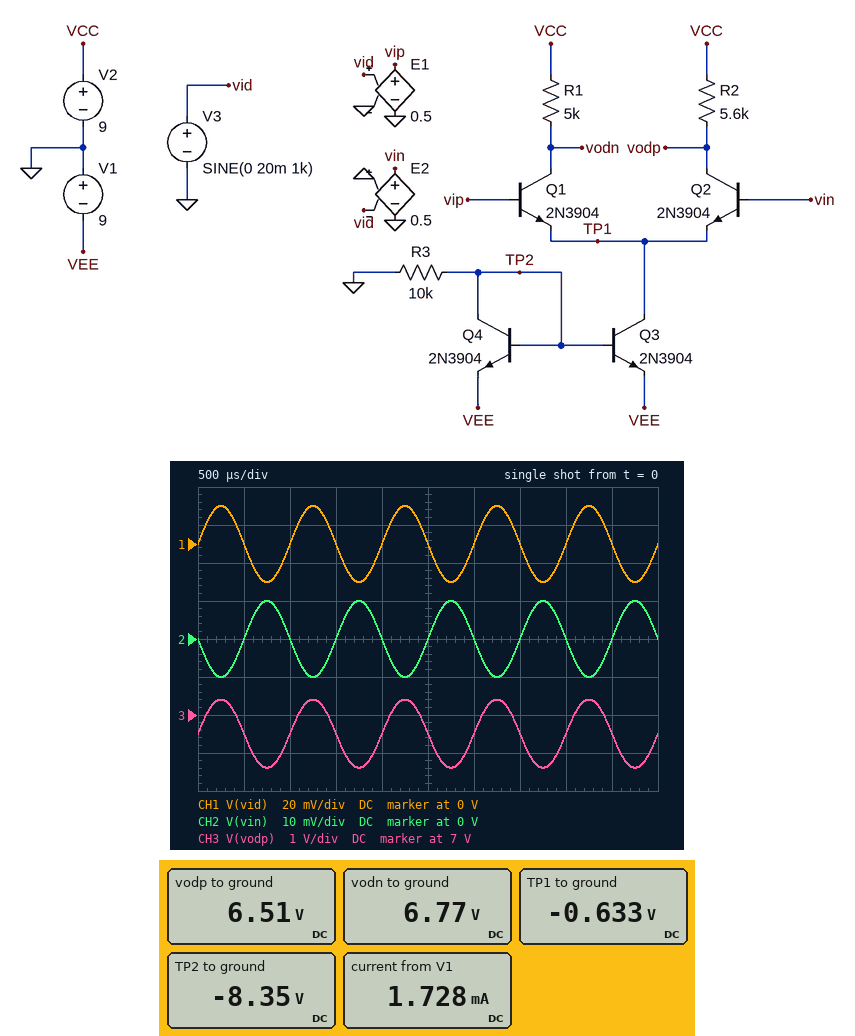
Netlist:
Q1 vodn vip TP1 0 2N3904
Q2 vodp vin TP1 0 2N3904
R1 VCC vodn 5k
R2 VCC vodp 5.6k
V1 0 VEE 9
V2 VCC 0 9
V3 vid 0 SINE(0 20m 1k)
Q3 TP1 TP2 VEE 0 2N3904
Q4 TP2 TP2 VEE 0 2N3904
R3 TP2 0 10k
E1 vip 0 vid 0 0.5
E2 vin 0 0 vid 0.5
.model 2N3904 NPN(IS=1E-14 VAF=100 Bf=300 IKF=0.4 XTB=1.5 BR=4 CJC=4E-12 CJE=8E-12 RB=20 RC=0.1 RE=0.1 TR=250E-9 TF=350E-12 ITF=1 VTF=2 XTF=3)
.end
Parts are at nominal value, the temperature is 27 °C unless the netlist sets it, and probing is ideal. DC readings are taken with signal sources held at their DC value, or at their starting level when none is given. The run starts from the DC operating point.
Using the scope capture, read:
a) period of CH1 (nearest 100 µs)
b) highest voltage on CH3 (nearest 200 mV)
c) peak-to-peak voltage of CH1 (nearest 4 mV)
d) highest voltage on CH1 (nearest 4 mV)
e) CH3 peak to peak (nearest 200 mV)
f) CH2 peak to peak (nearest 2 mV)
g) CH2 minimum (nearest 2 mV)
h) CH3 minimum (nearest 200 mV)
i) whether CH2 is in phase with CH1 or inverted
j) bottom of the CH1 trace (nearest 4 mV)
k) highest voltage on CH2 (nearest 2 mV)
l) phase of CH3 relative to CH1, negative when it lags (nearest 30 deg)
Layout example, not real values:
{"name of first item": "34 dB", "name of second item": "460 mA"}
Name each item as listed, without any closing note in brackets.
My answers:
{"period of CH1": "1.0 ms", "highest voltage on CH3": "7.4 V", "peak-to-peak voltage of CH1": "40 mV", "highest voltage on CH1": "20 mV", "CH3 peak to peak": "1.8 V", "CH2 peak to peak": "20 mV", "CH2 minimum": "-10 mV", "CH3 minimum": "5.6 V", "whether CH2 is in phase with CH1 or inverted": "inverted", "bottom of the CH1 trace": "-20 mV", "highest voltage on CH2": "10 mV", "phase of CH3 relative to CH1, negative when it lags": "0 deg"}
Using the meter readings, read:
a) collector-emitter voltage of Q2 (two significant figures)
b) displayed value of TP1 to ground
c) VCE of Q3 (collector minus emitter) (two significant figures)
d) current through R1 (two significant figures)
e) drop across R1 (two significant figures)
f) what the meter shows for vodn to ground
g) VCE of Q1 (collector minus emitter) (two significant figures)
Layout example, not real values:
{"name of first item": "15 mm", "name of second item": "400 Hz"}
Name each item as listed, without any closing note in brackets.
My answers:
{"collector-emitter voltage of Q2": "7.1 V", "displayed value of TP1 to ground": "-0.633 V", "VCE of Q3 (collector minus emitter)": "8.4 V", "current through R1": "450 µA", "drop across R1": "2.2 V", "what the meter shows for vodn to ground": "6.77 V", "VCE of Q1 (collector minus emitter)": "7.4 V"}
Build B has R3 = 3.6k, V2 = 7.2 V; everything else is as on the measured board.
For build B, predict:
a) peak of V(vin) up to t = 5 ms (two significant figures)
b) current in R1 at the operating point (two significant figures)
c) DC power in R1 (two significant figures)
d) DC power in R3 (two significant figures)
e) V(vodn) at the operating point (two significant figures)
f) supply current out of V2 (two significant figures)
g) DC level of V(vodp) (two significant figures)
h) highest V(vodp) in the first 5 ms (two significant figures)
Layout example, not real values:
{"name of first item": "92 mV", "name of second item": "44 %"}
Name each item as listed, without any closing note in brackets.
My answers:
{"peak of V(vin) up to t = 5 ms": "10 mV", "current in R1 at the operating point": "1.2 mA", "DC power in R1": "7.6 mW", "DC power in R3": "19 mW", "V(vodn) at the operating point": "1.0 V", "supply current out of V2": "2.5 mA", "DC level of V(vodp)": "330 mV", "highest V(vodp) in the first 5 ms": "2.4 V"}
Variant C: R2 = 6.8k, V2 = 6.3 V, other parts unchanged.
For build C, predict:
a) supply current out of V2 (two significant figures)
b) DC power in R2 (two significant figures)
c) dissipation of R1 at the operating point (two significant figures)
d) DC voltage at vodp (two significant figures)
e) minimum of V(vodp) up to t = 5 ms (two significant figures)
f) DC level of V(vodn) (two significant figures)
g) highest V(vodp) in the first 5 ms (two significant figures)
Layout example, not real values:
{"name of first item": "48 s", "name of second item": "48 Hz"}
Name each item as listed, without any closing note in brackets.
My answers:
{"supply current out of V2": "890 µA", "DC power in R2": "1.3 mW", "dissipation of R1 at the operating point": "1.0 mW", "DC voltage at vodp": "3.3 V", "minimum of V(vodp) up to t = 5 ms": "2.2 V", "DC level of V(vodn)": "4.1 V", "highest V(vodp) in the first 5 ms": "4.4 V"}
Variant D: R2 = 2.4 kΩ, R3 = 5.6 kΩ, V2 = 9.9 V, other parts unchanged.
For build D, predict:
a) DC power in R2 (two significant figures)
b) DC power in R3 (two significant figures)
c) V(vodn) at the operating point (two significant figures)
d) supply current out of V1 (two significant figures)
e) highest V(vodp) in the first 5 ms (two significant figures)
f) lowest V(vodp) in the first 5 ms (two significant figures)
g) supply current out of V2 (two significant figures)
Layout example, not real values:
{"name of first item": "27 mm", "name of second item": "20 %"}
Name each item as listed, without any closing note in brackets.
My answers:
{"DC power in R2": "1.5 mW", "DC power in R3": "12 mW", "V(vodn) at the operating point": "6.0 V", "supply current out of V1": "3.1 mA", "highest V(vodp) in the first 5 ms": "8.7 V", "lowest V(vodp) in the first 5 ms": "7.3 V", "supply current out of V2": "1.6 mA"}
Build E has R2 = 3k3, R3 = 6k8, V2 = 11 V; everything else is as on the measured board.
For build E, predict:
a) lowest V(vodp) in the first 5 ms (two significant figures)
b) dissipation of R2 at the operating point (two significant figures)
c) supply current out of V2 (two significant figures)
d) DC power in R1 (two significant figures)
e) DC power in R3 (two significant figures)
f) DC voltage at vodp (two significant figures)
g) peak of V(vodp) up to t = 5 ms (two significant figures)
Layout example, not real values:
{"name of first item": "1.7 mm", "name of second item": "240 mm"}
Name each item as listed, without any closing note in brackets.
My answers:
{"lowest V(vodp) in the first 5 ms": "8.1 V", "dissipation of R2 at the operating point": "1.4 mW", "supply current out of V2": "1.3 mA", "DC power in R1": "2.1 mW", "DC power in R3": "10 mW", "DC voltage at vodp": "8.8 V", "peak of V(vodp) up to t = 5 ms": "9.6 V"}
